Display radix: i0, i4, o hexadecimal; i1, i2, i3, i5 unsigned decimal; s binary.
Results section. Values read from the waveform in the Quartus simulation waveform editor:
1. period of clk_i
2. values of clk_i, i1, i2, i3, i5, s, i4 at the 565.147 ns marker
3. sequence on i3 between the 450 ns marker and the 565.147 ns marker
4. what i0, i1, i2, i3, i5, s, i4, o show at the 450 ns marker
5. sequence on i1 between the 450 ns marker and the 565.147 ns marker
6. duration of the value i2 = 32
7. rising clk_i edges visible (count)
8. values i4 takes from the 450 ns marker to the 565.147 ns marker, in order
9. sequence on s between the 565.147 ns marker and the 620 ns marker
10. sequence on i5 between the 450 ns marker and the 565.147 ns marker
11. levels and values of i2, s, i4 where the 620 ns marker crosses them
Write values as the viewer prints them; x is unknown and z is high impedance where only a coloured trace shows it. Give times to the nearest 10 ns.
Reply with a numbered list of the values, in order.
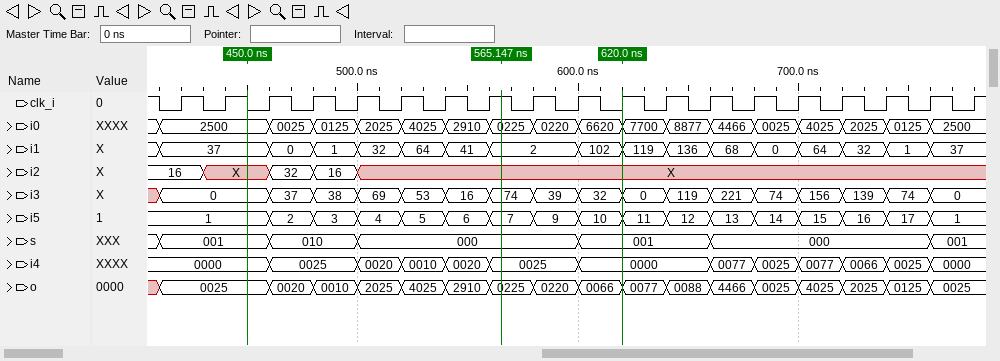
1. 20 ns
2. clk_i=1, i1=2, i2=X, i3=74, i5=7, s=000, i4=0025
3. 0, 37, 38, 69, 53, 16, 74
4. i0=2500, i1=37, i2=X, i3=0, i5=1, s=001, i4=0000, o=0025
5. 37, 0, 1, 32, 64, 41, 2
6. 20 ns
7. 19
8. 0000, 0025, 0020, 0010, 0020, 0025
9. 000, 001
10. 1, 2, 3, 4, 5, 6, 7
11. i2=X, s=001, i4=0000
